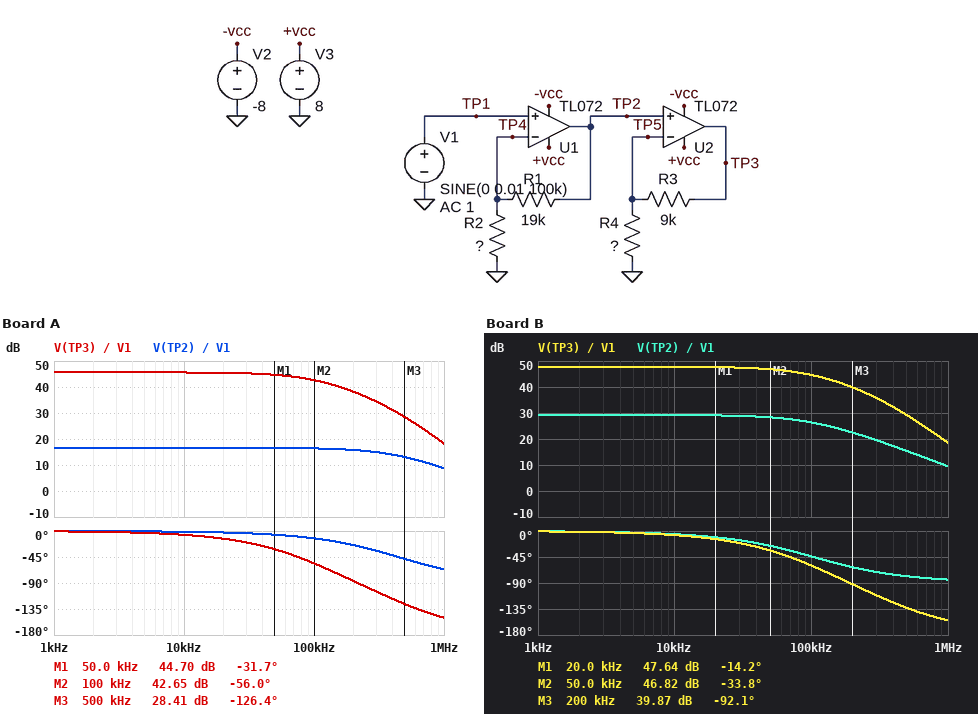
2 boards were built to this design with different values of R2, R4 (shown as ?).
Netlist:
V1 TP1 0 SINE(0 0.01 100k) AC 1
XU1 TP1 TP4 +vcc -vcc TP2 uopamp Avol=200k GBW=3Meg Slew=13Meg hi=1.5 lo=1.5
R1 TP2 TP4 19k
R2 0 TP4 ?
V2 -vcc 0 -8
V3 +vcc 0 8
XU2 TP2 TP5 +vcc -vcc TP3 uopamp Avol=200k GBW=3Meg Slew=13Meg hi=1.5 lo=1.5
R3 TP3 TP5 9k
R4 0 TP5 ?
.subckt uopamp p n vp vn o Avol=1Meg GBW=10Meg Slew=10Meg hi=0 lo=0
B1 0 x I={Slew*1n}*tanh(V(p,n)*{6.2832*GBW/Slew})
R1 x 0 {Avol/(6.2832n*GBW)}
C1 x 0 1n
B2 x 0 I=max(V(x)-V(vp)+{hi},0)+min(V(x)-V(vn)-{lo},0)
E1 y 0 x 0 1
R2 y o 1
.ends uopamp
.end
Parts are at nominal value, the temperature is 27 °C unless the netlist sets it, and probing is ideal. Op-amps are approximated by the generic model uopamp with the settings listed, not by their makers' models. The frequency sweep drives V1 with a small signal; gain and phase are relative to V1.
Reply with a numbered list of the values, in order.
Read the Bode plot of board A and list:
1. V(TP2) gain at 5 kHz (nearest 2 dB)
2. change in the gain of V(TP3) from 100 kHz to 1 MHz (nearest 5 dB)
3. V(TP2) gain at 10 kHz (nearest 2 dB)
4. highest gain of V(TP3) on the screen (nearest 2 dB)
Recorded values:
1. 16 dB
2. -25 dB
3. 16 dB
4. 46 dB
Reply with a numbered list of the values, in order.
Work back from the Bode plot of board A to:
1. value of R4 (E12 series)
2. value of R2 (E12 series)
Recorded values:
1. 330 Ω
2. 3.3 kΩ
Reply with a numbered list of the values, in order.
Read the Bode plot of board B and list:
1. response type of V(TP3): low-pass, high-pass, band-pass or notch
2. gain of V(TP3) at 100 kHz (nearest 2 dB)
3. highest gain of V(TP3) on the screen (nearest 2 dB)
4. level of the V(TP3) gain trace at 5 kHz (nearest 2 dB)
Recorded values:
1. low-pass
2. 44 dB
3. 48 dB
4. 48 dB
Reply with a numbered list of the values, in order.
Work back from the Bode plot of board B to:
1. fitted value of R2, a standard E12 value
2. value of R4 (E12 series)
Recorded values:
1. 680 Ω
2. 1.2 kΩ
